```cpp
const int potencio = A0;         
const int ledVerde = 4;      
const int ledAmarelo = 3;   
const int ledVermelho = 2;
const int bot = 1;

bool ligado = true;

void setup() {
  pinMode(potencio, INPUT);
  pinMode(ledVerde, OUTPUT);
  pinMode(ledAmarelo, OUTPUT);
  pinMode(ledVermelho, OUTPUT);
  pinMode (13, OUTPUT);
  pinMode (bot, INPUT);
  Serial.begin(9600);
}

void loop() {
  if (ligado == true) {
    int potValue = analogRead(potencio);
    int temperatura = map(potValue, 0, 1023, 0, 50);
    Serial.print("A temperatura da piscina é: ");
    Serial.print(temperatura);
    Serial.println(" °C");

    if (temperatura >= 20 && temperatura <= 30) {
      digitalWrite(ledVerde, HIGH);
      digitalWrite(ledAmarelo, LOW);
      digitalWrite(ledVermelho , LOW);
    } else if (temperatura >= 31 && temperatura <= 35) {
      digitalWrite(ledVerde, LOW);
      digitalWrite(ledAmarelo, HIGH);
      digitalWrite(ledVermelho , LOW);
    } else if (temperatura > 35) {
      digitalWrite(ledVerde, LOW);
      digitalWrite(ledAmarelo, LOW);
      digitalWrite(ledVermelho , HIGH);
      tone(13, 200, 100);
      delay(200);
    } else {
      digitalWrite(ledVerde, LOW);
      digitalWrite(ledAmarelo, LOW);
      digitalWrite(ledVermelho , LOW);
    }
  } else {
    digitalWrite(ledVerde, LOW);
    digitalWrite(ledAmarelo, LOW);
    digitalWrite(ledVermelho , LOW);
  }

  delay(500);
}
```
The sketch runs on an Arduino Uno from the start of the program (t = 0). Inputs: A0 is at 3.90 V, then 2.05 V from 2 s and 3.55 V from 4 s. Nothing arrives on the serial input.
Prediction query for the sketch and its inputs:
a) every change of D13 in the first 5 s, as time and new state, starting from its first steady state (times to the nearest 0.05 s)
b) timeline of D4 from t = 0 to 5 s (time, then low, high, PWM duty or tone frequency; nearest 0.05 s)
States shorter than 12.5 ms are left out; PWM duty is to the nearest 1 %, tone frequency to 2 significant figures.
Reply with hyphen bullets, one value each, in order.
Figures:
- 0 s tone 200 Hz; 0.1 s low; 0.7 s tone 200 Hz; 0.8 s low; 1.4 s tone 200 Hz; 1.5 s low
- 0 s low; 2.1 s high; 4.1 s low
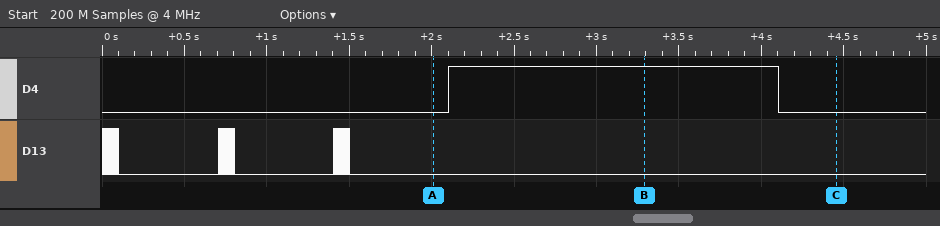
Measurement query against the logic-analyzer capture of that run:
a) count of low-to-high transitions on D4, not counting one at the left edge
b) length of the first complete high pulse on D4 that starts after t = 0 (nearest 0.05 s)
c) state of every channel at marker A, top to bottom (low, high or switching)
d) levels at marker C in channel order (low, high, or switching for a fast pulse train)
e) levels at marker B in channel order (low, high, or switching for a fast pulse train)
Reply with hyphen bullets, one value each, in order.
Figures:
- 1
- 2.00 s
- D4 low, D13 low
- D4 low, D13 low
- D4 high, D13 low
